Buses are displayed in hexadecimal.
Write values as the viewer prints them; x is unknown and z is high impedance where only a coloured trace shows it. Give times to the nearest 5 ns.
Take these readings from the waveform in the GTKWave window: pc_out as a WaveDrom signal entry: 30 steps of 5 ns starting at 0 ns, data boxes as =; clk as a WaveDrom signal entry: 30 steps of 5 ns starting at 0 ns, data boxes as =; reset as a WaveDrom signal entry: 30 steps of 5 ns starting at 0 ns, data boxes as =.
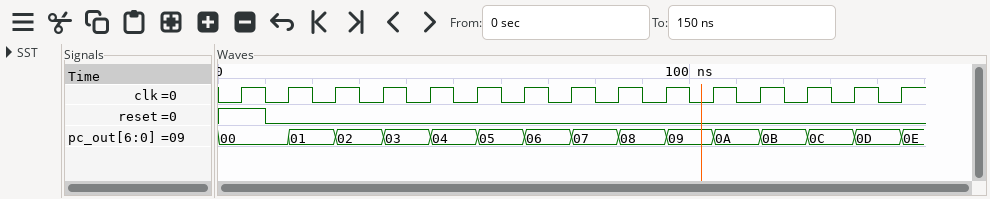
{name: 'pc_out', wave: '=..=.=.=.=.=.=.=.=.=.=.=.=.=.=', data: '00 01 02 03 04 05 06 07 08 09 0A 0B 0C 0D 0E'}
{name: 'clk', wave: '010101010101010101010101010101'}
{name: 'reset', wave: '1.0...........................'}
